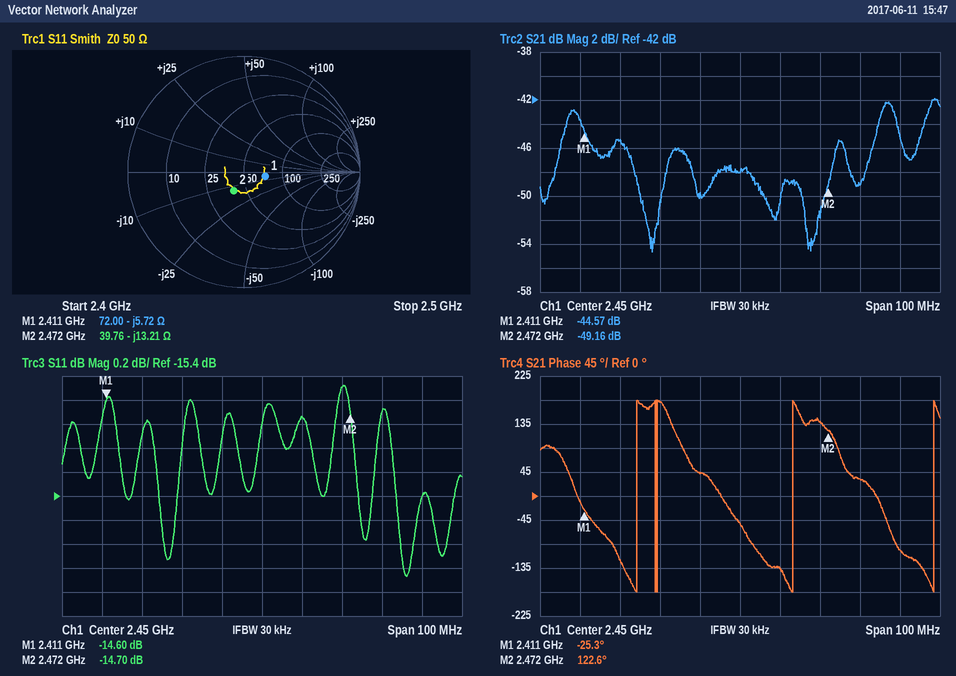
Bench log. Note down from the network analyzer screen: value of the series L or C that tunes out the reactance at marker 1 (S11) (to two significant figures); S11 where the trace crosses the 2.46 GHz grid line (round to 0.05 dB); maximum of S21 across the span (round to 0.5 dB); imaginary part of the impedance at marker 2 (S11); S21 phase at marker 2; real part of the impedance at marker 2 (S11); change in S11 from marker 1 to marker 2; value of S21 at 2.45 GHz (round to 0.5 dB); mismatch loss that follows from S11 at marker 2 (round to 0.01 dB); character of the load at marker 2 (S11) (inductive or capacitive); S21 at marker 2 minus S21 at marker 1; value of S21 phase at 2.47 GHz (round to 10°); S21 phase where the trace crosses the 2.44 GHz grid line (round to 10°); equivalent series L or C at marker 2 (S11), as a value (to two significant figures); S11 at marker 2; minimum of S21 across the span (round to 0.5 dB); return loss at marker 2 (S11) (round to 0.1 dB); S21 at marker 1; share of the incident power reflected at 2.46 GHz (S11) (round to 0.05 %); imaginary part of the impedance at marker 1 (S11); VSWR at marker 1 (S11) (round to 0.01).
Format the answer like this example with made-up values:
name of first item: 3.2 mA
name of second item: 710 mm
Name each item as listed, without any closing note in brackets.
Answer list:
value of the series L or C that tunes out the reactance at marker 1 (S11): 380 pH
S11 where the trace crosses the 2.46 GHz grid line: -14.75 dB
maximum of S21 across the span: -42.0 dB
imaginary part of the impedance at marker 2: -13.21 Ω
S21 phase at marker 2: 122.6°
real part of the impedance at marker 2: 39.76 Ω
change in S11 from marker 1 to marker 2: -0.10 dB
value of S21 at 2.45 GHz: -48.0 dB
mismatch loss that follows from S11 at marker 2: 0.15 dB
character of the load at marker 2 (S11): capacitive
S21 at marker 2 minus S21 at marker 1: -4.59 dB
value of S21 phase at 2.47 GHz: 140°
S21 phase where the trace crosses the 2.44 GHz grid line: 40°
equivalent series L or C at marker 2 (S11), as a value: 4.9 pF
S11 at marker 2: -14.70 dB
minimum of S21 across the span: -54.5 dB
return loss at marker 2 (S11): 14.7 dB
S21 at marker 1: -44.57 dB
share of the incident power reflected at 2.46 GHz (S11): 3.35 %
imaginary part of the impedance at marker 1: -5.72 Ω
VSWR at marker 1 (S11): 1.46
